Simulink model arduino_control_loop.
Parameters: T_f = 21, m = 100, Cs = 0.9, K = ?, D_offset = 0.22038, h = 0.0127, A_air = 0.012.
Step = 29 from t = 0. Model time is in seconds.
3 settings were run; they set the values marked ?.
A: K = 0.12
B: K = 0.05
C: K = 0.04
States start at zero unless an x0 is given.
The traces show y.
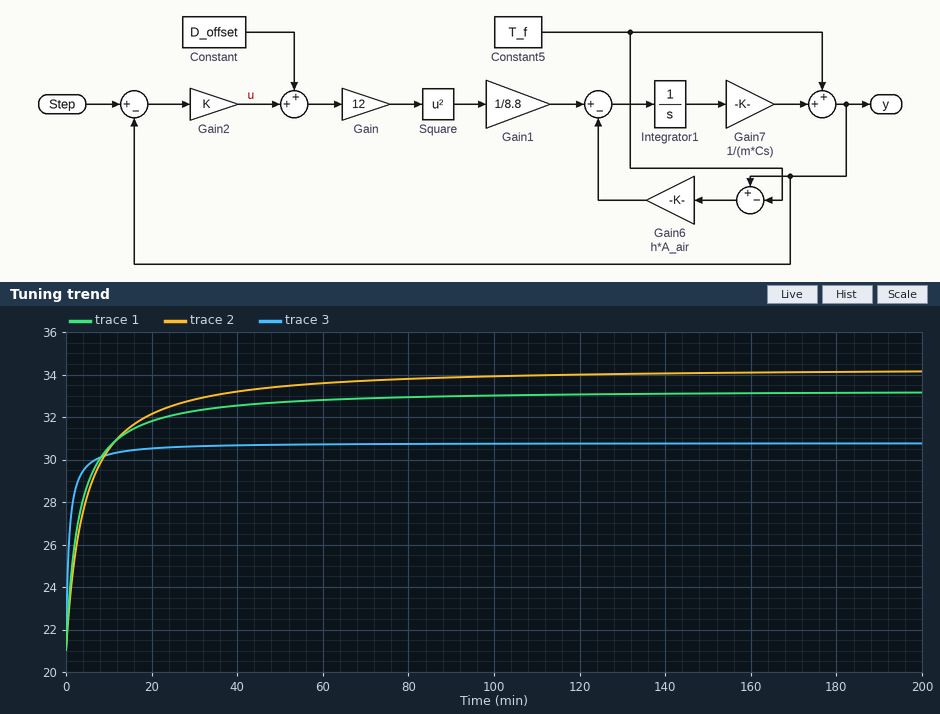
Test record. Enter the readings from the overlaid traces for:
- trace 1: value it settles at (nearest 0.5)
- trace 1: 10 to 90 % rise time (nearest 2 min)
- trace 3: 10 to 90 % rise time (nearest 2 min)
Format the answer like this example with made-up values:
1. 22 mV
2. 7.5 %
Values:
1. 33.0
2. 22 min
3. 6 min
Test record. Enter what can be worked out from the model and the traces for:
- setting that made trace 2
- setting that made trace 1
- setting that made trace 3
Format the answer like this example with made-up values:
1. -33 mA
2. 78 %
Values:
1. C
2. B
3. A
